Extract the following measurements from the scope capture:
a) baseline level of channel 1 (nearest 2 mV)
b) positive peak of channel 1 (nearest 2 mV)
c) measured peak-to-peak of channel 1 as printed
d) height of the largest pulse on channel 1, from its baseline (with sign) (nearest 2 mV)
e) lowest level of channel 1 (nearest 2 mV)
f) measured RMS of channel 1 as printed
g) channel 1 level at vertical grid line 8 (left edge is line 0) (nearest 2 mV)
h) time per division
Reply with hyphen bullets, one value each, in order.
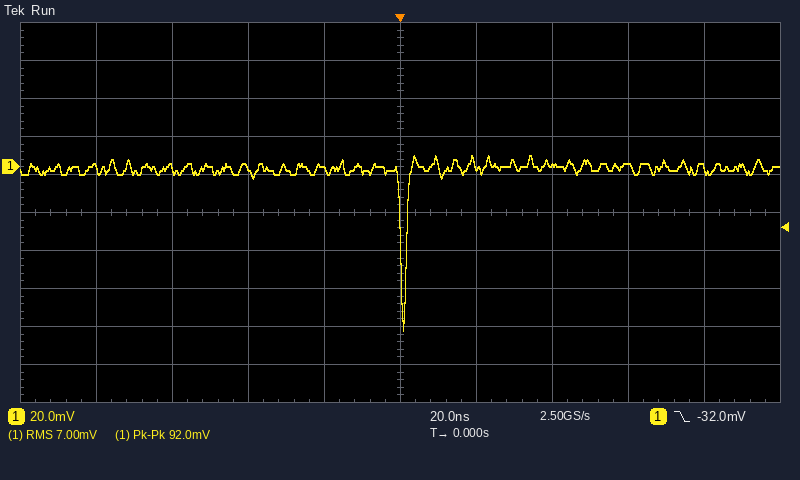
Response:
- 0 mV
- 6 mV
- 92.0 mV
- -86 mV
- -86 mV
- 7.00 mV
- 0 mV
- 20 ns
